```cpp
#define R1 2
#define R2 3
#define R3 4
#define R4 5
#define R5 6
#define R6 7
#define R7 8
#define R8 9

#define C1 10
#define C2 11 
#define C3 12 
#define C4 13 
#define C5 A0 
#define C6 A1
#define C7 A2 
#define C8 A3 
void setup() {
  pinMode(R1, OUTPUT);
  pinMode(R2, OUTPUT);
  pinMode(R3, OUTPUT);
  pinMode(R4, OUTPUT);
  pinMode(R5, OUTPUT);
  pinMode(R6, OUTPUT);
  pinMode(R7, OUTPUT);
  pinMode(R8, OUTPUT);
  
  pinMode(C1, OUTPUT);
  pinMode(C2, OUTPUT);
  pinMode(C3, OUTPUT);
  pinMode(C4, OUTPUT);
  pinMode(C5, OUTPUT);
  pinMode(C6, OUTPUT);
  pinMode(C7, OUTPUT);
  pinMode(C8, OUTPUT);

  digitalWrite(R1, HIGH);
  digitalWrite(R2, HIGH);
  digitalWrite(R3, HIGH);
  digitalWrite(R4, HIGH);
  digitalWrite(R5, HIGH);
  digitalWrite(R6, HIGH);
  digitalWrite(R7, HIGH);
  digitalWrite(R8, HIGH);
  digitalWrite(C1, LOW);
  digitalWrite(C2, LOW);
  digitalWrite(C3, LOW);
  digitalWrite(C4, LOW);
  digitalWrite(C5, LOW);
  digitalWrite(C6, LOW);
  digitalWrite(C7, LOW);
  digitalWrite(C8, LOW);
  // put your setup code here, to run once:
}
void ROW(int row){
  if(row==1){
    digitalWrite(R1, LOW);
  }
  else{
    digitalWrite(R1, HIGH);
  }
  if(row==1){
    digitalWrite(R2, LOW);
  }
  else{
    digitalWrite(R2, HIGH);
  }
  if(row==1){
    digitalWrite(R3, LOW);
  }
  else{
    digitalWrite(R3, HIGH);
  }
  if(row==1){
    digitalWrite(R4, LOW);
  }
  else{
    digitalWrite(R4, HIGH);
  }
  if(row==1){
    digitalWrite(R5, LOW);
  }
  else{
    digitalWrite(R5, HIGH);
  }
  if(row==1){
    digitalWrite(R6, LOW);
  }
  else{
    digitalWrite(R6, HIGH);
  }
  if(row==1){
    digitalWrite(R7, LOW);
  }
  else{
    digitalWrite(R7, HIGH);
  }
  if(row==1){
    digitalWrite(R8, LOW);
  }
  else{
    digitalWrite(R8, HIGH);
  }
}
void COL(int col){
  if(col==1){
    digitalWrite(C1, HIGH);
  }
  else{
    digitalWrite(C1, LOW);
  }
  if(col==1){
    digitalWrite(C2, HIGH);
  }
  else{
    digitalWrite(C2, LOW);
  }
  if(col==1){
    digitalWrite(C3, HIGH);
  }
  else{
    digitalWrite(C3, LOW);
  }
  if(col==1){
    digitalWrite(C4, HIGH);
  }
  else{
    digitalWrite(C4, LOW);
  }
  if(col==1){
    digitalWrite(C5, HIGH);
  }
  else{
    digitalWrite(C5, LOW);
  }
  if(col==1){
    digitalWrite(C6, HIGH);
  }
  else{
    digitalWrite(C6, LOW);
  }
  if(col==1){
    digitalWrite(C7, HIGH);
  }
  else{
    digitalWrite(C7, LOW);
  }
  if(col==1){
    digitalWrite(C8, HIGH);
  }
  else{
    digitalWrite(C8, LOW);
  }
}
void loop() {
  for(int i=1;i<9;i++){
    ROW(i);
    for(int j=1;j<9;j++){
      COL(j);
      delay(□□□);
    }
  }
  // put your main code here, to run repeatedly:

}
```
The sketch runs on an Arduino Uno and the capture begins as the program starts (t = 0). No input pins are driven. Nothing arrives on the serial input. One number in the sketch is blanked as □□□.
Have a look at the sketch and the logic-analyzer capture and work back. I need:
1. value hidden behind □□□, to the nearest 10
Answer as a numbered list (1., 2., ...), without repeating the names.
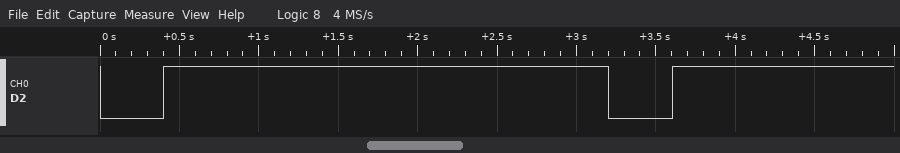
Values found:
1. 50
